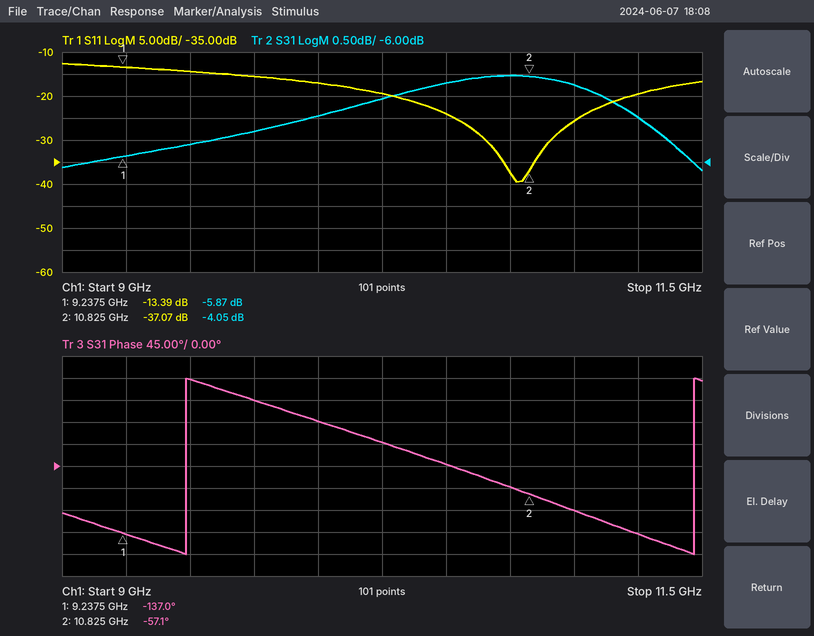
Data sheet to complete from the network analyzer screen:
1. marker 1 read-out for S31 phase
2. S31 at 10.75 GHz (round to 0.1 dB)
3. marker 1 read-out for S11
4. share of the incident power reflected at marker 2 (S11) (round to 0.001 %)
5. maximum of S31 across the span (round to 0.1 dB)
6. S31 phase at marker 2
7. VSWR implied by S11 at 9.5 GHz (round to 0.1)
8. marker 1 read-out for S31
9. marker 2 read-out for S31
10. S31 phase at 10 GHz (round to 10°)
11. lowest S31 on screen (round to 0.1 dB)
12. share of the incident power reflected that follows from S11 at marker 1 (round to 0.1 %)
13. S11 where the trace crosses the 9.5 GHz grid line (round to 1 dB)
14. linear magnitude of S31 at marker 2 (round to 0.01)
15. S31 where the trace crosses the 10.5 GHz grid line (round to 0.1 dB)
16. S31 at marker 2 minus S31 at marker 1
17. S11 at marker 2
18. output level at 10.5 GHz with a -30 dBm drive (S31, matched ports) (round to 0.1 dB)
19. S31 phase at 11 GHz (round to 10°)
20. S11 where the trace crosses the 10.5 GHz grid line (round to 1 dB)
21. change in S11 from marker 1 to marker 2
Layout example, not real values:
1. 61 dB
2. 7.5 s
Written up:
1. -137.0°
2. -4.0 dB
3. -13.39 dB
4. 0.020 %
5. -4.0 dB
6. -57.1°
7. 1.5
8. -5.87 dB
9. -4.05 dB
10. 90°
11. -6.2 dB
12. 4.6 %
13. -14 dB
14. 0.63
15. -4.2 dB
16. 1.82 dB
17. -37.07 dB
18. -34.2 dBm
19. -90°
20. -24 dB
21. -23.68 dB
